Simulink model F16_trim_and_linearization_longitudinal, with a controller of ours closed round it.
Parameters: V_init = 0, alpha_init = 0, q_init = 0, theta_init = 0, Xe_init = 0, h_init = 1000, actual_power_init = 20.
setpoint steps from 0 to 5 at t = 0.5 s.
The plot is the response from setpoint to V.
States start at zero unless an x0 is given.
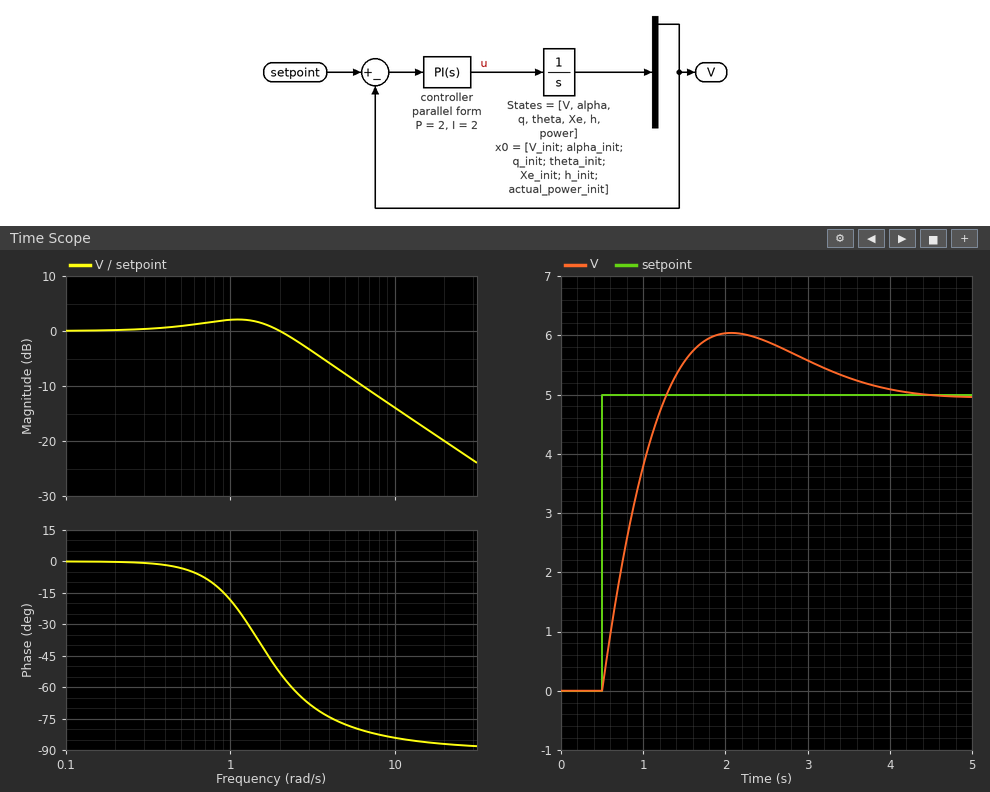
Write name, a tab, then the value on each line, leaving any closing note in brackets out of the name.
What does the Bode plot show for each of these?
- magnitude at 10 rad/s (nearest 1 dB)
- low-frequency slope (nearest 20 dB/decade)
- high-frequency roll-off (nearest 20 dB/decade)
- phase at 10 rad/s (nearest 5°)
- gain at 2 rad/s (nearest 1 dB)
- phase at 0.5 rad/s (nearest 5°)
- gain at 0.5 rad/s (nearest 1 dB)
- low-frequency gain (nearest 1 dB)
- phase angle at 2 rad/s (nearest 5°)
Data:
magnitude at 10 rad/s	-14 dB
low-frequency slope	0 dB/decade
high-frequency roll-off	-20 dB/decade
phase at 10 rad/s	-85°
gain at 2 rad/s	0 dB
phase at 0.5 rad/s	-5°
gain at 0.5 rad/s	1 dB
low-frequency gain	0 dB
phase angle at 2 rad/s	-55°
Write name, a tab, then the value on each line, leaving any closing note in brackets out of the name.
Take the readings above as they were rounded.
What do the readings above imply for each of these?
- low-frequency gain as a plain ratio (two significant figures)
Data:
low-frequency gain as a plain ratio	1.0
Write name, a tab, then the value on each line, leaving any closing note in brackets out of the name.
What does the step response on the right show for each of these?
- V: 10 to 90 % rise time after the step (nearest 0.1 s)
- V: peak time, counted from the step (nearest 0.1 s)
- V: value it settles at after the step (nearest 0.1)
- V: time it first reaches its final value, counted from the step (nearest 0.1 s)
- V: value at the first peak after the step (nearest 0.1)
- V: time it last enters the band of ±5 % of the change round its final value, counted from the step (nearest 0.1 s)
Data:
V: 10 to 90 % rise time after the step	0.6 s
V: peak time, counted from the step	1.6 s
V: value it settles at after the step	5.0
V: time it first reaches its final value, counted from the step	0.8 s
V: value at the first peak after the step	6.0
V: time it last enters the band of ±5 % of the change round its final value, counted from the step	3.1 s
